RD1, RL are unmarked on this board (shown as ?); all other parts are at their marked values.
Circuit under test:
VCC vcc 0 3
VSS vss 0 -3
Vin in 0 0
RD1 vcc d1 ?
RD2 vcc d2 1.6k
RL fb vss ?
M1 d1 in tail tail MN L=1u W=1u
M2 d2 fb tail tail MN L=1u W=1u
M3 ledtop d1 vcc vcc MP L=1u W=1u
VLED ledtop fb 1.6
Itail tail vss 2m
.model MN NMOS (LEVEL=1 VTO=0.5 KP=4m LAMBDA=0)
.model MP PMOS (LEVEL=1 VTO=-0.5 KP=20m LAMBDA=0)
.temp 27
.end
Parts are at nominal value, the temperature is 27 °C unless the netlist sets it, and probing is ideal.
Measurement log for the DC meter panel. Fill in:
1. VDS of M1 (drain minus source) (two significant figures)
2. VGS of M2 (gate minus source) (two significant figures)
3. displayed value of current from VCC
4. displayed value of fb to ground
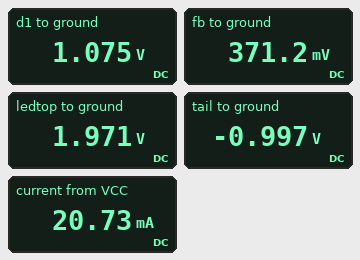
2.1 V
1.4 V
20.73 mA
371.2 mV
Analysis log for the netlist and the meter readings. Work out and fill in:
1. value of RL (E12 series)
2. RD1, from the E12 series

180 Ω
3.9 kΩ
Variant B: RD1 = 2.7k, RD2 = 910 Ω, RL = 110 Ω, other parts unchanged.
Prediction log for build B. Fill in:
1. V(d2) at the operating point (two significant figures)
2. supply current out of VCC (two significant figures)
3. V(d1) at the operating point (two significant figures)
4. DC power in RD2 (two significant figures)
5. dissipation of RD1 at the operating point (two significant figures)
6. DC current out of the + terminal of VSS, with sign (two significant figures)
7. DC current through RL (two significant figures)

1.9 V
30 mA
750 mV
1.2 mW
1.9 mW
-30 mA
28 mA
